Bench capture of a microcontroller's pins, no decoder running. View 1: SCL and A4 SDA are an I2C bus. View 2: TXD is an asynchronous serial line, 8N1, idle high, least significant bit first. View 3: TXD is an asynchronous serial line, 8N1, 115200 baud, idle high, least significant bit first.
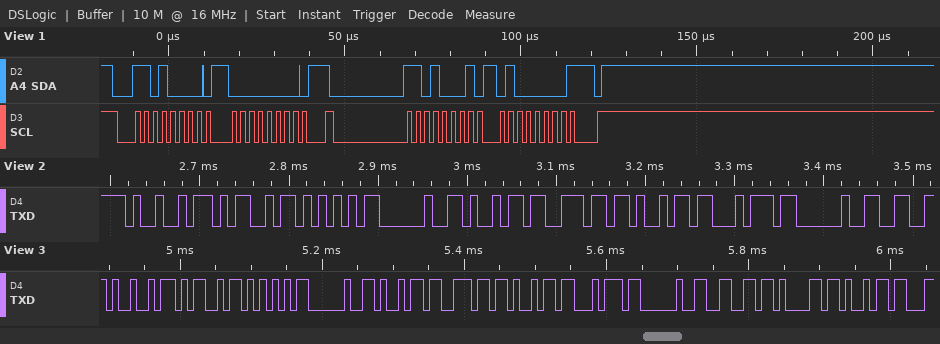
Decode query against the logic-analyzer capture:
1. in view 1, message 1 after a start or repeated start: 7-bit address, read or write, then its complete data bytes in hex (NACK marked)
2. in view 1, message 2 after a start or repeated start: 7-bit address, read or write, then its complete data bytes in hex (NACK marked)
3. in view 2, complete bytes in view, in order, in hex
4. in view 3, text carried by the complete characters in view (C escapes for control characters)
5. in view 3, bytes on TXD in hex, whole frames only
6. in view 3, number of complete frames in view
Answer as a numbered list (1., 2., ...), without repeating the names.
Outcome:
1. 0x68 write: 00
2. 0x68 read: 40 NACK
3. 49 4D 55 20 69 6E 69 74 20
4. "IMU init fai"
5. 0x49 0x4D 0x55 0x20 0x69 0x6E 0x69 0x74 0x20 0x66 0x61 0x69
6. 12
